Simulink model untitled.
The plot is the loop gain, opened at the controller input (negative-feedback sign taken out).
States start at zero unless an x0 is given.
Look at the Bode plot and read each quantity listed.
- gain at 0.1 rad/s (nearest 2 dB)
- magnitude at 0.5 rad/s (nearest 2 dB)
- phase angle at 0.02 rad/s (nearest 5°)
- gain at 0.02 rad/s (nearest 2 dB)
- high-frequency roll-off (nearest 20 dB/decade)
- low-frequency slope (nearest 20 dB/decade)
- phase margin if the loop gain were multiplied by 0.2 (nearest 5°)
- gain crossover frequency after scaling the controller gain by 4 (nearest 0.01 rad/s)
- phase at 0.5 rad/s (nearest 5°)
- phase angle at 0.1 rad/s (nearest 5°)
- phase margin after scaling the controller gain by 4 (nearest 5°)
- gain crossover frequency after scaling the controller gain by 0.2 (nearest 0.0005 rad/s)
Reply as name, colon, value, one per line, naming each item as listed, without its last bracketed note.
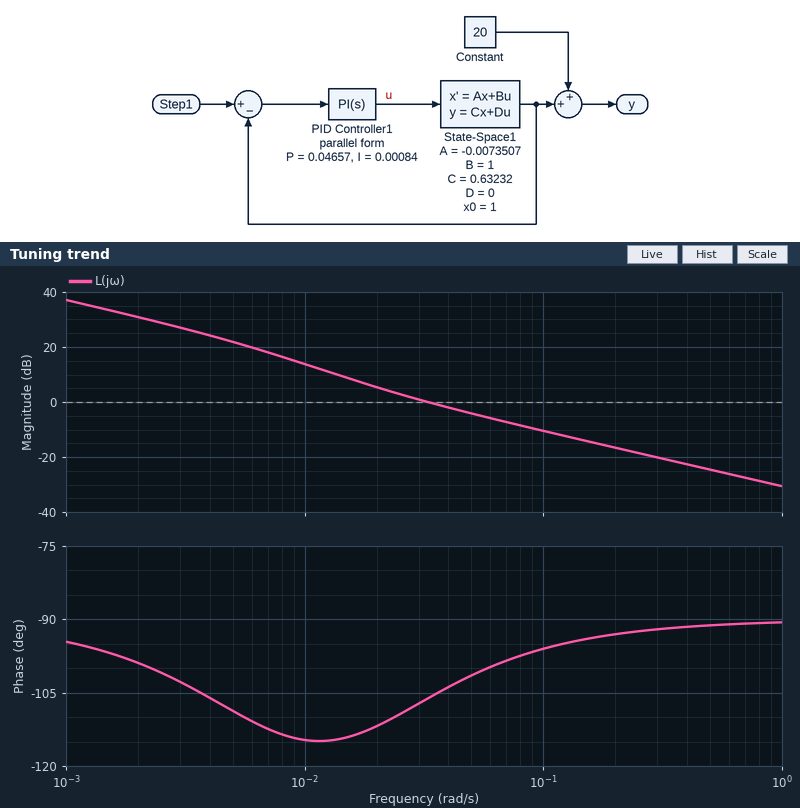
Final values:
gain at 0.1 rad/s: -10 dB
magnitude at 0.5 rad/s: -24 dB
phase angle at 0.02 rad/s: -110°
gain at 0.02 rad/s: 6 dB
high-frequency roll-off: -20 dB/decade
low-frequency slope: -20 dB/decade
phase margin if the loop gain were multiplied by 0.2: 65°
gain crossover frequency after scaling the controller gain by 4: 0.12 rad/s
phase at 0.5 rad/s: -90°
phase angle at 0.1 rad/s: -95°
phase margin after scaling the controller gain by 4: 85°
gain crossover frequency after scaling the controller gain by 0.2: 0.0100 rad/s
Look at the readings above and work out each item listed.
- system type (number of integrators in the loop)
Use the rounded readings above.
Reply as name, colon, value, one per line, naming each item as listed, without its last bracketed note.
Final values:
system type: 1
